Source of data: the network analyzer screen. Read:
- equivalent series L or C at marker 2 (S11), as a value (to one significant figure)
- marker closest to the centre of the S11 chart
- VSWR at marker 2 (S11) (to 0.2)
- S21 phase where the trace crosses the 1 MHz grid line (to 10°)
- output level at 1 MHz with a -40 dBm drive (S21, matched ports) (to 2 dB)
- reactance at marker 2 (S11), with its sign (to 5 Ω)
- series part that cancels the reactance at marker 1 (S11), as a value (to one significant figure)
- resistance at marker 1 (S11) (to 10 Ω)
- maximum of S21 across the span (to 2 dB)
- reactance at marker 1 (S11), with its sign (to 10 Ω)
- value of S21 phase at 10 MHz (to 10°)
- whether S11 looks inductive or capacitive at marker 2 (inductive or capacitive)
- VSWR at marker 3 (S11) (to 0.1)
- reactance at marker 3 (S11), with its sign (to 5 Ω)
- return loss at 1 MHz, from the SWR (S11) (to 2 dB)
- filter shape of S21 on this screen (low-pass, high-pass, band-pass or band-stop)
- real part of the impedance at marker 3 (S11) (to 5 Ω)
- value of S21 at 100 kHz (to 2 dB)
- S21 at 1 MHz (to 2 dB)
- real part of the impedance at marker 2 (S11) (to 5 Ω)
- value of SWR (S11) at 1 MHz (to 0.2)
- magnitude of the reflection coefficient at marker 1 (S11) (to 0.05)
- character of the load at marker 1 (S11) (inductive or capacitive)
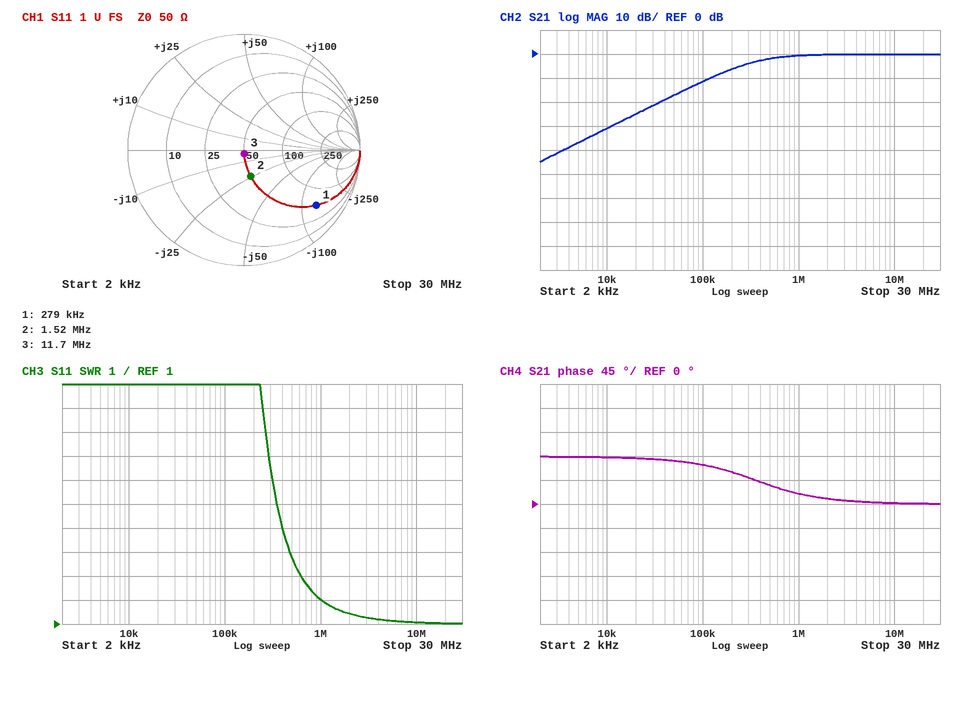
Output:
4 nF
marker 3
1.6
20°
-40 dBm
-25 Ω
70 µH
50 Ω
0 dB
-130 Ω
0°
capacitive
1.1
-5 Ω
10 dB
high-pass
50 Ω
-12 dB
0 dB
50 Ω
2.0
0.80
capacitive
